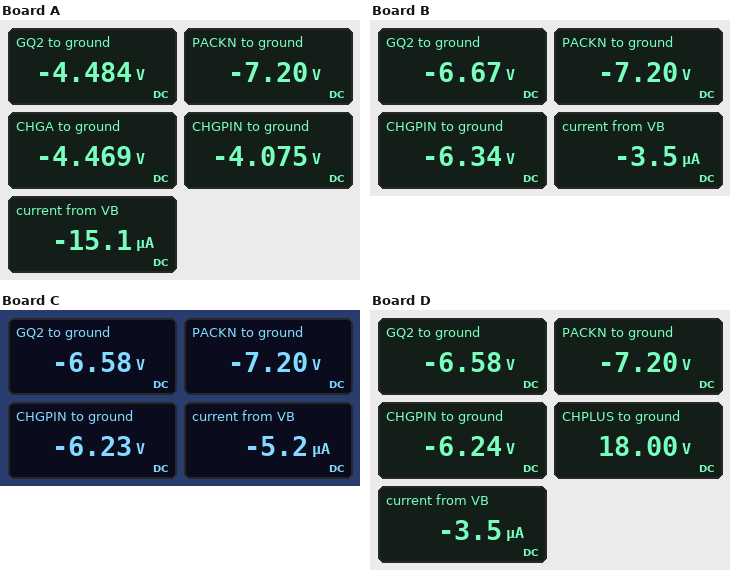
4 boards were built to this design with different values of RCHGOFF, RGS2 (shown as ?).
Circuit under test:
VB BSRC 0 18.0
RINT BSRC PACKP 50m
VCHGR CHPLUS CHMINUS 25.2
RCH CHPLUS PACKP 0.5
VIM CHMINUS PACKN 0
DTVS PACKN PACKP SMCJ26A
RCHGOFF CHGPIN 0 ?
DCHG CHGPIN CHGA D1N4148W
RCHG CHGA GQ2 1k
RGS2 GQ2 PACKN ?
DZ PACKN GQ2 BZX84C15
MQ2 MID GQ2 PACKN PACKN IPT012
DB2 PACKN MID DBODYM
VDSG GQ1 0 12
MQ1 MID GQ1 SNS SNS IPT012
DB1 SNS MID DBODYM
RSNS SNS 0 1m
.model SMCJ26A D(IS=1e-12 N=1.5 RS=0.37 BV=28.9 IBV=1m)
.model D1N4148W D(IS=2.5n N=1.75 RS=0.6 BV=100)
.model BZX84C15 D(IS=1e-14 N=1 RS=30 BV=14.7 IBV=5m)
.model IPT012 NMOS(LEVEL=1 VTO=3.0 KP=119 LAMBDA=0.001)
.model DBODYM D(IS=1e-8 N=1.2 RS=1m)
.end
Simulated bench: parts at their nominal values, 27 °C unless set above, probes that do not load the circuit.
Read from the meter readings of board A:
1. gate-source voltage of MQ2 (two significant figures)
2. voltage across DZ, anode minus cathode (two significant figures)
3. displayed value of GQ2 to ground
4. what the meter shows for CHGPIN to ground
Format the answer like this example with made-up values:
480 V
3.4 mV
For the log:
2.7 V
-2.7 V
-4.484 V
-4.075 V
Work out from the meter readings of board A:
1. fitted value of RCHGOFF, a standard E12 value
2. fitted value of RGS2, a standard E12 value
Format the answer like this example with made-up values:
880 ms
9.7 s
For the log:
270 kΩ
180 kΩ
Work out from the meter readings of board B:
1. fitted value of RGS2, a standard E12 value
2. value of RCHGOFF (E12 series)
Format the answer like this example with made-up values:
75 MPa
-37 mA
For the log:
150 kΩ
1.8 MΩ
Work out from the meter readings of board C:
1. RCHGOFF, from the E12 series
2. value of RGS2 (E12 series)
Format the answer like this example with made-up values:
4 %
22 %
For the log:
1.2 MΩ
120 kΩ
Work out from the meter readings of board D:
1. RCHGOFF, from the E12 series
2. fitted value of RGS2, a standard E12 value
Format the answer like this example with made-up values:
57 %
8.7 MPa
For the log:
1.8 MΩ
180 kΩ
